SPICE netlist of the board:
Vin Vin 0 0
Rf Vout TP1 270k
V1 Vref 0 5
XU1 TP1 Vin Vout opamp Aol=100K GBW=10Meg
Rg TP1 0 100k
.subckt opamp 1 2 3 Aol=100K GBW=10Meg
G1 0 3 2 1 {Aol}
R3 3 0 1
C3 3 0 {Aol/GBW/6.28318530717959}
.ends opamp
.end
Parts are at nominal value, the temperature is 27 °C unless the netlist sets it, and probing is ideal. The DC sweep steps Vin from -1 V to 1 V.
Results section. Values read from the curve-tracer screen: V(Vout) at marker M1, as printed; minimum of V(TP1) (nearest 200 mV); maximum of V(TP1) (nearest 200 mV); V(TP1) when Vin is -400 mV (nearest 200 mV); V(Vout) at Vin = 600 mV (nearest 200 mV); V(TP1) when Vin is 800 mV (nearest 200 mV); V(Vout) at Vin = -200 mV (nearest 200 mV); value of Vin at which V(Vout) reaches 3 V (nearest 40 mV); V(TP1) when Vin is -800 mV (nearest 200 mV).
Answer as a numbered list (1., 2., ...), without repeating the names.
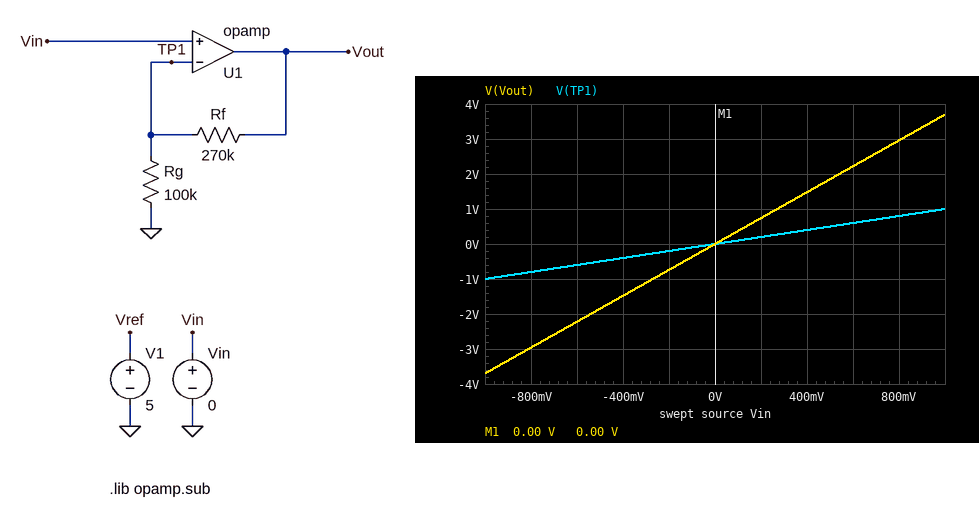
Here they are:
1. 0.00 V
2. -1.0 V
3. 1.0 V
4. -400 mV
5. 2.2 V
6. 800 mV
7. -800 mV
8. 800 mV
9. -800 mV
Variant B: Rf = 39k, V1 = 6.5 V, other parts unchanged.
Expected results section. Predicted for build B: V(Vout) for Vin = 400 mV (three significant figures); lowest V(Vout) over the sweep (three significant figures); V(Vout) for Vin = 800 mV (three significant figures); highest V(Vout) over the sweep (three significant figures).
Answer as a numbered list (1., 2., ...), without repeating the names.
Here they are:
1. 556 mV
2. -1.39 V
3. 1.11 V
4. 1.39 V
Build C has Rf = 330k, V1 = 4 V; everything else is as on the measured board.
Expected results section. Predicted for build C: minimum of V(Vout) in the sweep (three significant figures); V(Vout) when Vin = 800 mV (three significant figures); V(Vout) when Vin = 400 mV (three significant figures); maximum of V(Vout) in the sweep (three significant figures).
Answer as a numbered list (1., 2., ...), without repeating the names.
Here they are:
1. -4.30 V
2. 3.44 V
3. 1.72 V
4. 4.30 V
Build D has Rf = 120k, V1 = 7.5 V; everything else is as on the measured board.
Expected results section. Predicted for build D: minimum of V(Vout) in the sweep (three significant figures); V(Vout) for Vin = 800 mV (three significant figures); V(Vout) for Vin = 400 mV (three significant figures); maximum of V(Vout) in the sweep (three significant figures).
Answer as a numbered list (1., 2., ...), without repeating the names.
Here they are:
1. -2.20 V
2. 1.76 V
3. 880 mV
4. 2.20 V
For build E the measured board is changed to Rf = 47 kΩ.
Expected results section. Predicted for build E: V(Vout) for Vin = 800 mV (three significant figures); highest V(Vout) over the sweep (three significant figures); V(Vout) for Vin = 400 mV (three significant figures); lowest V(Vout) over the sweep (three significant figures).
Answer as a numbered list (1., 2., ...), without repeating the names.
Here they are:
1. 1.18 V
2. 1.47 V
3. 588 mV
4. -1.47 V
